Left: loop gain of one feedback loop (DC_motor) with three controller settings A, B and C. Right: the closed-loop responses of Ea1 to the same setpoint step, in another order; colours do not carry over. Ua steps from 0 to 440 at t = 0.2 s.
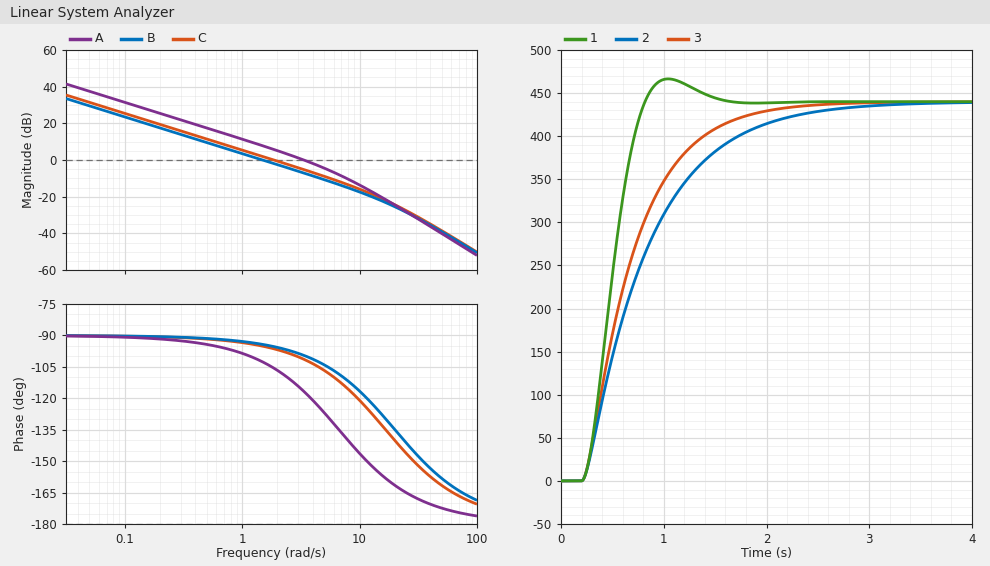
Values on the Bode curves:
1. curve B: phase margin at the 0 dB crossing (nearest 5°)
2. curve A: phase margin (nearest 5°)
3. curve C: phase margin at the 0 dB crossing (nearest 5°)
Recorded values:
85°
65°
85°
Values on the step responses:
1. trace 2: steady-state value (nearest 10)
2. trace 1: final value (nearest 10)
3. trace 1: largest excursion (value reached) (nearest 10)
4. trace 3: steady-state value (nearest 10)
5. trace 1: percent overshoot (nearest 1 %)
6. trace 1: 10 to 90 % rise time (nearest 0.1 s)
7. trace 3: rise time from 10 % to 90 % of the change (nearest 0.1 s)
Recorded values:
440
440
470
440
6 %
0.4 s
1.0 s
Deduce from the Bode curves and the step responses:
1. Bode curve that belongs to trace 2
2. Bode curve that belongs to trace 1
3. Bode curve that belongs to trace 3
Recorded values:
B
A
C
